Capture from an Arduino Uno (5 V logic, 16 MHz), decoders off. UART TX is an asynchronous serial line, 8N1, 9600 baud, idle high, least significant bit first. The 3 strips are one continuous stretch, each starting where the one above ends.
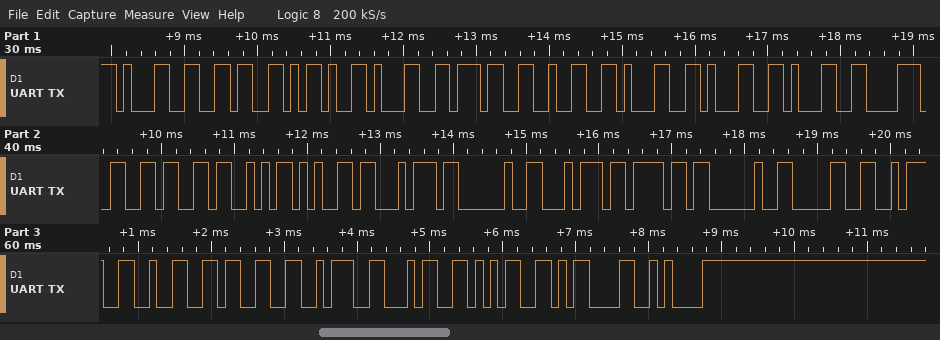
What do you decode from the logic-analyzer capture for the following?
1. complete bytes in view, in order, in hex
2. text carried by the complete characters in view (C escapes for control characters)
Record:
31 36 2D 31 37 32 31 31 31 38 36 53 65 74 20 74 6F 20 30 3A 32 33 3A 34 35 0D 0A
"16-17211186Set to 0:23:45\r\n"
